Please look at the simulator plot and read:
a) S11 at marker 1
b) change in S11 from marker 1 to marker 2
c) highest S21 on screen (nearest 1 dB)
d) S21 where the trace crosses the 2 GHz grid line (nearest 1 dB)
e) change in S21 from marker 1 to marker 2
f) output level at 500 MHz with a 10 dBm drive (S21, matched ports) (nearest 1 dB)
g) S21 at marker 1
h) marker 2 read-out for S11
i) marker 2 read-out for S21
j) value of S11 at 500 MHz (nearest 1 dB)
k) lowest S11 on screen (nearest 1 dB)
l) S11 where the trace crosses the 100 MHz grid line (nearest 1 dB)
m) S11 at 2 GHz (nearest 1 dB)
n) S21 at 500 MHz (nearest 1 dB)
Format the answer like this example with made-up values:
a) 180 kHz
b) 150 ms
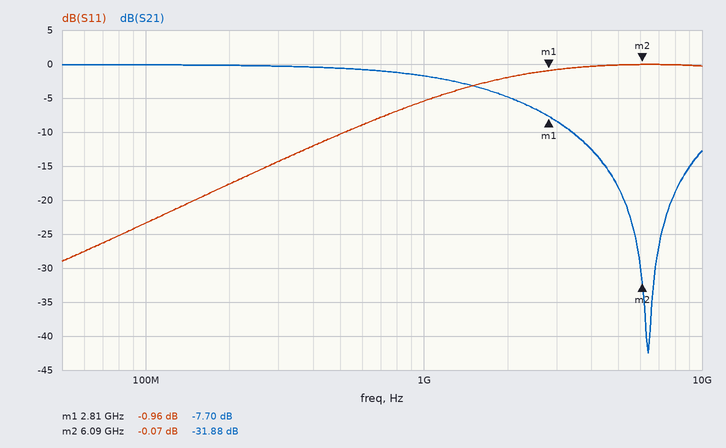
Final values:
a) -0.96 dB
b) 0.89 dB
c) 0 dB
d) -5 dB
e) -24.18 dB
f) 9 dBm
g) -7.70 dB
h) -0.07 dB
i) -31.88 dB
j) -10 dB
k) -29 dB
l) -23 dB
m) -2 dB
n) -1 dB
